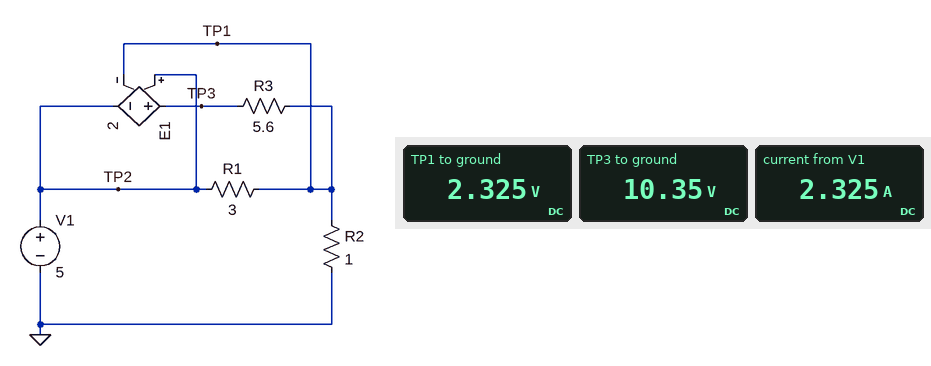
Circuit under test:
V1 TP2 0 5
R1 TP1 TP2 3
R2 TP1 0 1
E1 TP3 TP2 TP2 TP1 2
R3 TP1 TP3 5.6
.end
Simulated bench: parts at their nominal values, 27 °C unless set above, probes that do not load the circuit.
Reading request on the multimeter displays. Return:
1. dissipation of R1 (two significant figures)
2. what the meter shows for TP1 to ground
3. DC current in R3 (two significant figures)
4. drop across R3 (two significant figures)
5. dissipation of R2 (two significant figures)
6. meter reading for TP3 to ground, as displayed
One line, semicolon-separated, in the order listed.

2.4 W; 2.325 V; 1.4 A; 8.0 V; 5.4 W; 10.35 V
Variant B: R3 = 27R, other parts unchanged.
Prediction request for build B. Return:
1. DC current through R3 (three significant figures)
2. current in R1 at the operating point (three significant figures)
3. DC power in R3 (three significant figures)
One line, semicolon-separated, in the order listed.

385 mA; 1.15 A; 3.99 W
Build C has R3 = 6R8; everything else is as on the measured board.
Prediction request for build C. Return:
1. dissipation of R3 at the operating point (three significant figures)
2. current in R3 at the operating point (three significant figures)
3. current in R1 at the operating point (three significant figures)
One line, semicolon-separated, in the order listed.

10.5 W; 1.24 A; 939 mA
